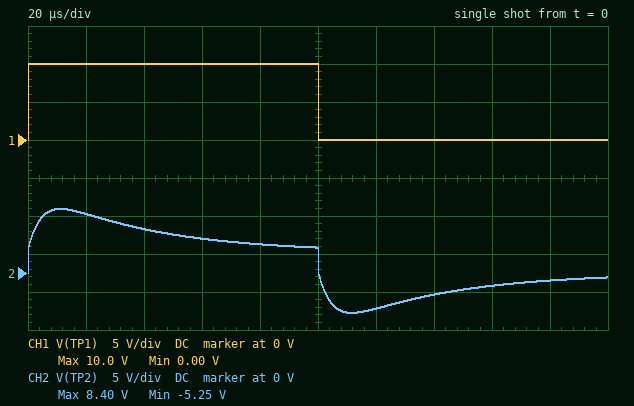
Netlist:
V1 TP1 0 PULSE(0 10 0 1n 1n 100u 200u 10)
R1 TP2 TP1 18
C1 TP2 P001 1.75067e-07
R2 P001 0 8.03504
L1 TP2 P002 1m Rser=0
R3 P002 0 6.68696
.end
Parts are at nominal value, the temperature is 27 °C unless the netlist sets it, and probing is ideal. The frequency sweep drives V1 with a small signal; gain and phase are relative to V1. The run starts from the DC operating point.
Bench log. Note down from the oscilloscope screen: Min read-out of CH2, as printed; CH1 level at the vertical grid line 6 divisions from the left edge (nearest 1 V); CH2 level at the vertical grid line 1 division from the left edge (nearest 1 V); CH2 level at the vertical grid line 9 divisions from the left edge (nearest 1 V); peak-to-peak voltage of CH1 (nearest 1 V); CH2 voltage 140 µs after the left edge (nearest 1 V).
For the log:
-5.25 V
0 V
8 V
-1 V
10 V
-3 V
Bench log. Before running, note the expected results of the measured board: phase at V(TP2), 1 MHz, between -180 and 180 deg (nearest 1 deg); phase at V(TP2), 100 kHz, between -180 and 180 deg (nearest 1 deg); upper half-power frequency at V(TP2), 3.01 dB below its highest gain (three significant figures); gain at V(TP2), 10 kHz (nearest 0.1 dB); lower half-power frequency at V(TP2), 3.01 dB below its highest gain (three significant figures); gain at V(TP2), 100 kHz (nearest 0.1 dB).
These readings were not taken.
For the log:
-4 deg
-29 deg
44.6 kHz
-0.4 dB
3.17 kHz
-7.1 dB
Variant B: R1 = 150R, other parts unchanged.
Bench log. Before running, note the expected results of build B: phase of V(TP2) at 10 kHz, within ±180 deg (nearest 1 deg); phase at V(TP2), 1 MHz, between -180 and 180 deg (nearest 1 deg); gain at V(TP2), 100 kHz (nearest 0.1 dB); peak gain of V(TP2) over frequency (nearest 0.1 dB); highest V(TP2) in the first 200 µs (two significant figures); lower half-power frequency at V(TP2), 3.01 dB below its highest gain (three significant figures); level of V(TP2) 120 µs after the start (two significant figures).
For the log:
27 deg
-6 deg
-22.2 dB
-2.8 dB
3.4 V
8.61 kHz
-2.7 V
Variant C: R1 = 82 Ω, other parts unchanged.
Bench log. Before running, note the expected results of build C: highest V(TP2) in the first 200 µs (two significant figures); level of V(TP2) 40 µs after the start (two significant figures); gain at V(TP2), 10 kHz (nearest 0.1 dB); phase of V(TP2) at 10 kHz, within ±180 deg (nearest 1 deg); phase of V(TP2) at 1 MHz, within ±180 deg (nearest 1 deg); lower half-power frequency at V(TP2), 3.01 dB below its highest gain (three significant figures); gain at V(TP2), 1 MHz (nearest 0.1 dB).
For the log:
4.9 V
1.8 V
-2.1 dB
18 deg
-6 deg
7.25 kHz
-20.9 dB
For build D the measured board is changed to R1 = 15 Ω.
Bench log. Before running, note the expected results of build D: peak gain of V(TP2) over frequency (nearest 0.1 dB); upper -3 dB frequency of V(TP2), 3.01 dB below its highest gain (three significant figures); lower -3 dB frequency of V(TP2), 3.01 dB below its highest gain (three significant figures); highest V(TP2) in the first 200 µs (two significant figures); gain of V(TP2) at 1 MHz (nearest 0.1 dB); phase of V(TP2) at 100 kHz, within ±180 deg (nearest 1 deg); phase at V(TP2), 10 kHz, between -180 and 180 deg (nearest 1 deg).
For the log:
-0.3 dB
50.9 kHz
2.78 kHz
8.7 V
-9.1 dB
-26 deg
4 deg
